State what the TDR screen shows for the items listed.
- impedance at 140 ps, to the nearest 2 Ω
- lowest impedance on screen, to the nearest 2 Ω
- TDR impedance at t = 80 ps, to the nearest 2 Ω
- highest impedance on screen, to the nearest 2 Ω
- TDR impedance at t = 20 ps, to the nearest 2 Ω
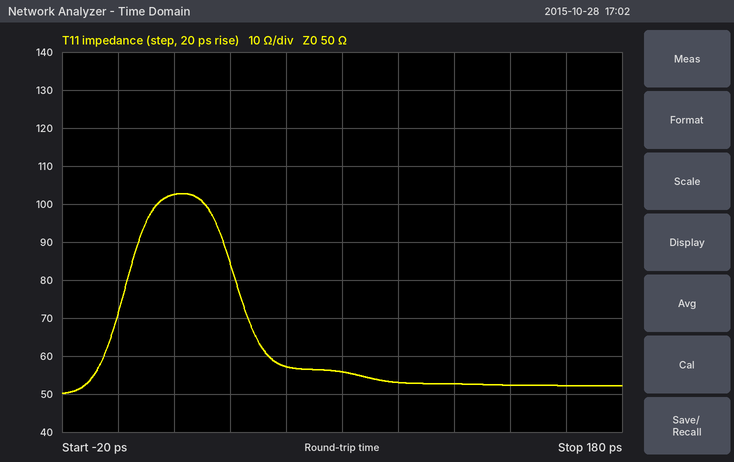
52 Ω
50 Ω
56 Ω
102 Ω
102 Ω
